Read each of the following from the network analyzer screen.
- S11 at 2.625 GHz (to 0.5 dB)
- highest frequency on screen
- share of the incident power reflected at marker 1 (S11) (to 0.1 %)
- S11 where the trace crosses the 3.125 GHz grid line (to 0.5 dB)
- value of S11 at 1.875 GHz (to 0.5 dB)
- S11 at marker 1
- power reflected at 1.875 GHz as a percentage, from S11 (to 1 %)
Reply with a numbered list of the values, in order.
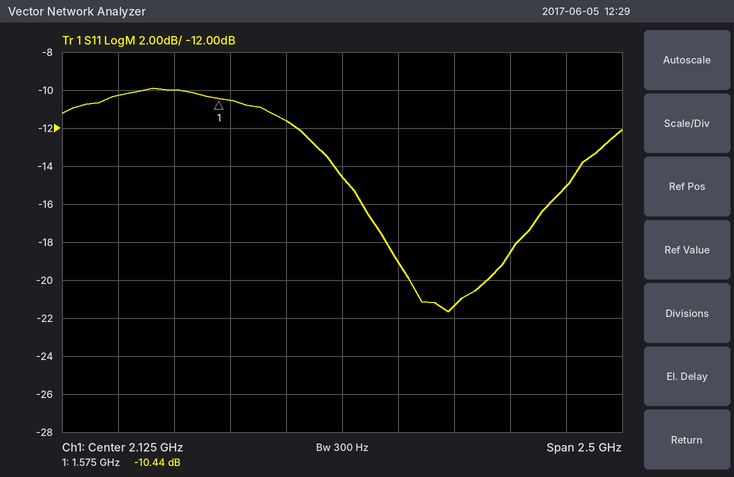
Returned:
1. -21.5 dB
2. 3.375 GHz
3. 9.0 %
4. -15.0 dB
5. -11.5 dB
6. -10.44 dB
7. 7 %
